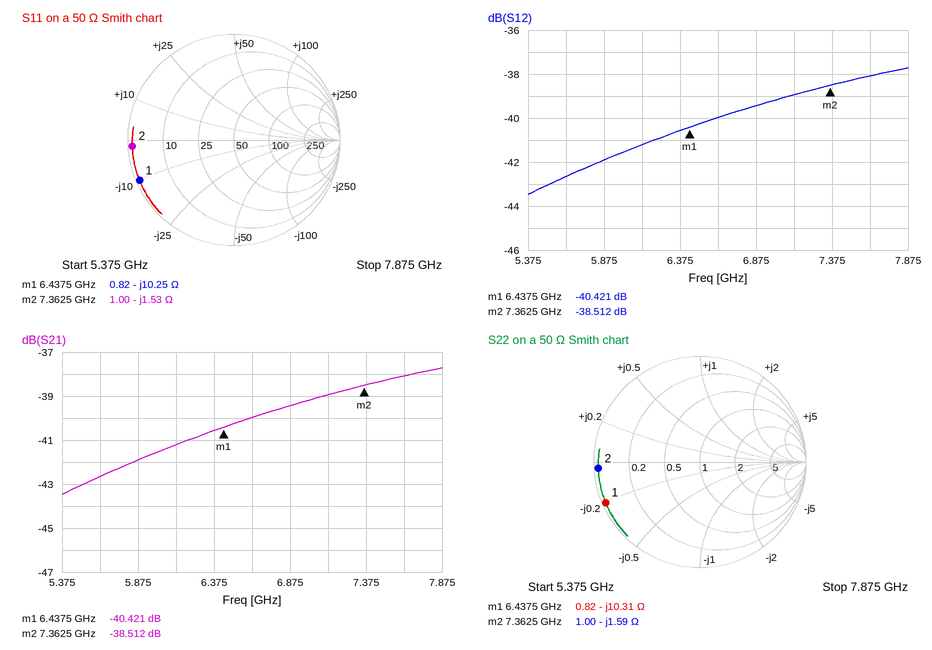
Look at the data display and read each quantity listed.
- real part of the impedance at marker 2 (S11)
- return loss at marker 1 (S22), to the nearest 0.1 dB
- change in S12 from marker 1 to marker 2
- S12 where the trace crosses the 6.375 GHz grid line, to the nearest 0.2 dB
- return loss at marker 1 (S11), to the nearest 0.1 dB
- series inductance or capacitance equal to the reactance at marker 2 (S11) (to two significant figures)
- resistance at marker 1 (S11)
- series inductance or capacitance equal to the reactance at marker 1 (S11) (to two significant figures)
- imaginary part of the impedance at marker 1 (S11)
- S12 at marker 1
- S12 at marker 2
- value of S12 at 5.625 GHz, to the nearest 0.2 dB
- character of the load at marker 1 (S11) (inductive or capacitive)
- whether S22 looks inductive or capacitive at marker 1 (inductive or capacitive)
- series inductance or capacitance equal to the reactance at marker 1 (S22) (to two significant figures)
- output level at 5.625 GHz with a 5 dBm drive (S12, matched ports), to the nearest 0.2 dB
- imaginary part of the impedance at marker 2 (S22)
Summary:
1.00 Ω
0.3 dB
1.909 dB
-40.6 dB
0.3 dB
14 pF
0.82 Ω
2.4 pF
-10.25 Ω
-40.421 dB
-38.512 dB
-42.6 dB
capacitive
capacitive
2.4 pF
-37.6 dBm
-1.59 Ω
